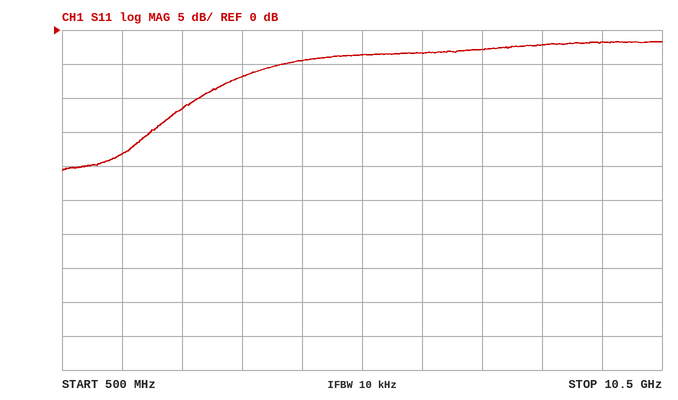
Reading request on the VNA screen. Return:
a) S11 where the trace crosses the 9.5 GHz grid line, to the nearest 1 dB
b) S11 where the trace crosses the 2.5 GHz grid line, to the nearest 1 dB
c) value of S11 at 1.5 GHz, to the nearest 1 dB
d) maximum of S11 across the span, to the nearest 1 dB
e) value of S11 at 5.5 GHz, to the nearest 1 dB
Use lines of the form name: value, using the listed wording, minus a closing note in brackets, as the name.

S11 where the trace crosses the 9.5 GHz grid line, to the nearest 1 dB: -2 dB
S11 where the trace crosses the 2.5 GHz grid line, to the nearest 1 dB: -12 dB
value of S11 at 1.5 GHz, to the nearest 1 dB: -18 dB
maximum of S11 across the span, to the nearest 1 dB: -2 dB
value of S11 at 5.5 GHz, to the nearest 1 dB: -4 dB
